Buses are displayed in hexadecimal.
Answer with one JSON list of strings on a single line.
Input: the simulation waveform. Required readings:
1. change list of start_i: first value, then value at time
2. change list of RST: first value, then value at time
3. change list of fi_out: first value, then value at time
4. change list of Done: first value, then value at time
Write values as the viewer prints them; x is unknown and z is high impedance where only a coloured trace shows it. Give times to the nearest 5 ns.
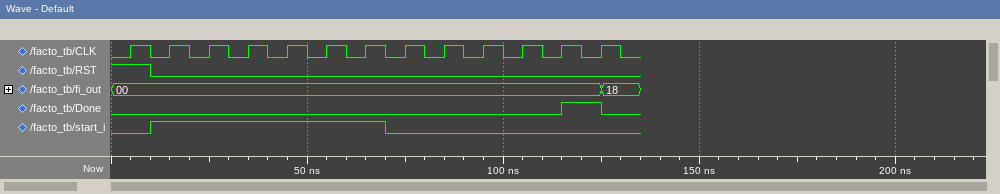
["0, 1 at 10 ns, 0 at 70 ns", "1, 0 at 10 ns", "00, 18 at 125 ns", "0, 1 at 115 ns, 0 at 125 ns"]
